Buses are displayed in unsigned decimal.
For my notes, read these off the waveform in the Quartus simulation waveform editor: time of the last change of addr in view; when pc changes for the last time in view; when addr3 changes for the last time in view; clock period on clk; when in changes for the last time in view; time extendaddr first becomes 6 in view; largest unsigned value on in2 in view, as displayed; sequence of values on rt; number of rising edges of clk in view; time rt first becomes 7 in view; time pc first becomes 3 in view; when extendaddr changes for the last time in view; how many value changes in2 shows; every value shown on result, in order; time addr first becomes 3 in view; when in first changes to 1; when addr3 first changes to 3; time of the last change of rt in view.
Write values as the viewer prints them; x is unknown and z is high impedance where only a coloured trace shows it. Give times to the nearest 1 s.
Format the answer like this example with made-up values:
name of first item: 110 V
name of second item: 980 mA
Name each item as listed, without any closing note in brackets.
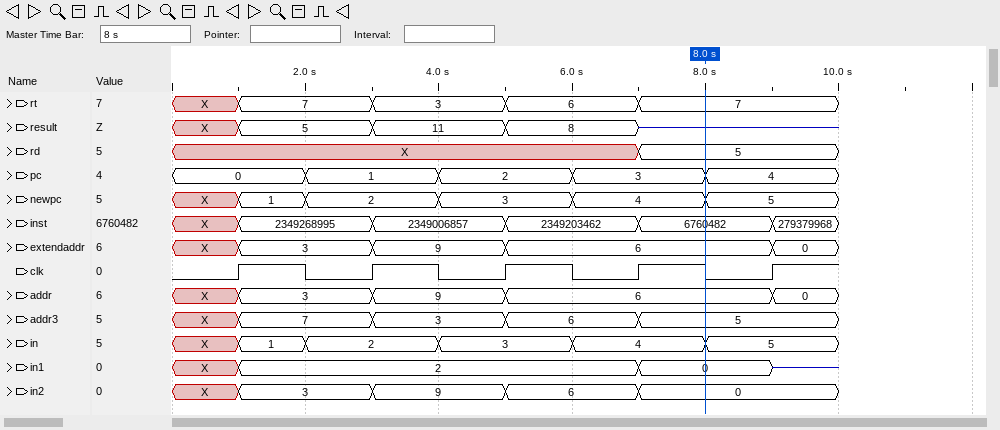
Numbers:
time of the last change of addr in view: 9 s
when pc changes for the last time in view: 8 s
when addr3 changes for the last time in view: 7 s
clock period on clk: 2 s
when in changes for the last time in view: 8 s
time extendaddr first becomes 6 in view: 5 s
largest unsigned value on in2 in view, as displayed: 9
sequence of values on rt: X, 7, 3, 6, 7
number of rising edges of clk in view: 5
time rt first becomes 7 in view: 1 s
time pc first becomes 3 in view: 6 s
when extendaddr changes for the last time in view: 9 s
how many value changes in2 shows: 4
every value shown on result, in order: X, 5, 11, 8, z
time addr first becomes 3 in view: 1 s
when in first changes to 1: 1 s
when addr3 first changes to 3: 3 s
time of the last change of rt in view: 7 s
